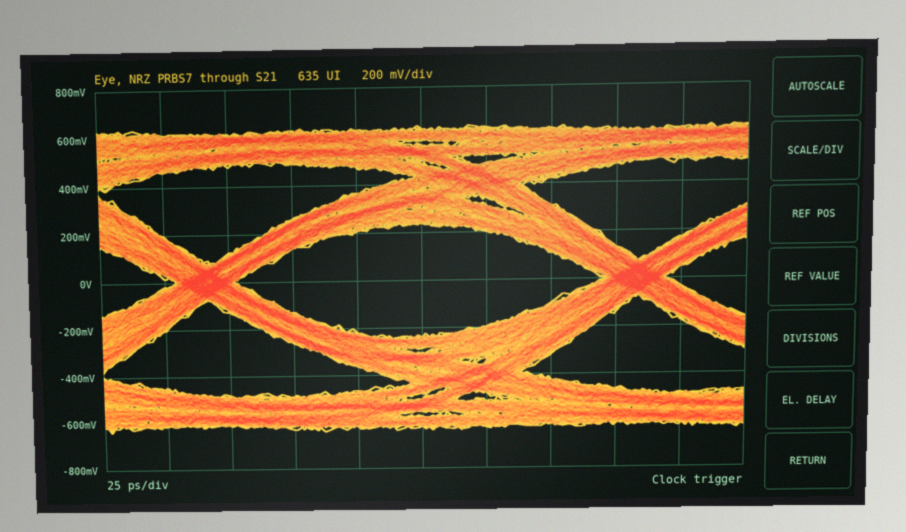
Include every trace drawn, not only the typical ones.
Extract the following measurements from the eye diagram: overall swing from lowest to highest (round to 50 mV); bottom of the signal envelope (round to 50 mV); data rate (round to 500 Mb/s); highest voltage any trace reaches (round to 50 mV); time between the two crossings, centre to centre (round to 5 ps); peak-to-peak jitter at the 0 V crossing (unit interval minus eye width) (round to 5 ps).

1.30 V
-650 mV
6.0 Gb/s
650 mV
165 ps
25 ps
